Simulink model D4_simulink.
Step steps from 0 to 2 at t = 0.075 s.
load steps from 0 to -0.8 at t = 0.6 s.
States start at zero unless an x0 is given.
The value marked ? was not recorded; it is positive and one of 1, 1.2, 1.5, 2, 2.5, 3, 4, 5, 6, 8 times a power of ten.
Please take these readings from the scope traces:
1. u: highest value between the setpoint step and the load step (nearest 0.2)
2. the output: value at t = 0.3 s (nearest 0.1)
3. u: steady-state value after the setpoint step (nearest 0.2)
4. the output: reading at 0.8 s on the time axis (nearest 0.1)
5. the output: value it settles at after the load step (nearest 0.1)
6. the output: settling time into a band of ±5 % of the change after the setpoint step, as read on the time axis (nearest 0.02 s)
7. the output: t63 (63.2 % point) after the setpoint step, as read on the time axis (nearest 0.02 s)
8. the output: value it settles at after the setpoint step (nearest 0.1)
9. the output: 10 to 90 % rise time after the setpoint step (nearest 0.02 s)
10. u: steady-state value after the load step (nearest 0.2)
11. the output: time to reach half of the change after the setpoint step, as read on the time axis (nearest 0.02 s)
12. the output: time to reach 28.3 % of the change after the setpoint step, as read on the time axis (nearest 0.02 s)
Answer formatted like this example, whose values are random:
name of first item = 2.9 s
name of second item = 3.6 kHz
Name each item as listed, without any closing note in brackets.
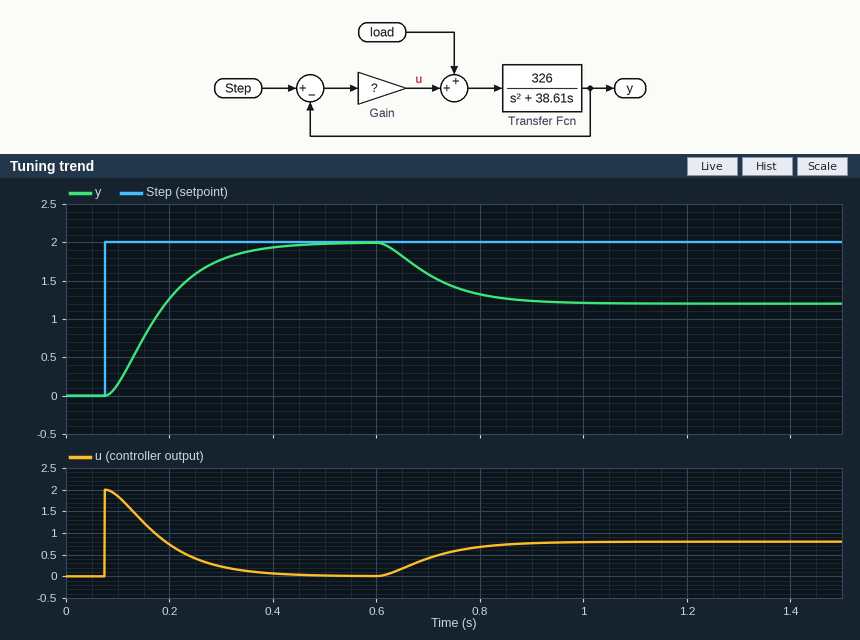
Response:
u: highest value between the setpoint step and the load step = 2.0
the output: value at t = 0.3 s = 1.8
u: steady-state value after the setpoint step = 0.0
the output: reading at 0.8 s on the time axis = 1.3
the output: value it settles at after the load step = 1.2
the output: settling time into a band of ±5 % of the change after the setpoint step, as read on the time axis = 0.36 s
the output: t63 (63.2 % point) after the setpoint step, as read on the time axis = 0.20 s
the output: value it settles at after the setpoint step = 2.0
the output: 10 to 90 % rise time after the setpoint step = 0.20 s
u: steady-state value after the load step = 0.8
the output: time to reach half of the change after the setpoint step, as read on the time axis = 0.18 s
the output: time to reach 28.3 % of the change after the setpoint step, as read on the time axis = 0.14 s
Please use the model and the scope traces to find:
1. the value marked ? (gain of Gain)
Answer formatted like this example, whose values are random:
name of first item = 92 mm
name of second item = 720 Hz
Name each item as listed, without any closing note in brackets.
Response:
the value marked ? = 1
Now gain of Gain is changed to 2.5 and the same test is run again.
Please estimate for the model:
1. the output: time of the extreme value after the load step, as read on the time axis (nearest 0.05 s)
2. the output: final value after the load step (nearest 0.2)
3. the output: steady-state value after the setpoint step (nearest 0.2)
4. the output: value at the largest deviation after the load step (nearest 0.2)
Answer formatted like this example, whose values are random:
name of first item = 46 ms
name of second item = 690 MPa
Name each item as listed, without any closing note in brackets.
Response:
the output: time of the extreme value after the load step, as read on the time axis = 0.75 s
the output: final value after the load step = 1.6
the output: steady-state value after the setpoint step = 2.0
the output: value at the largest deviation after the load step = 1.6
